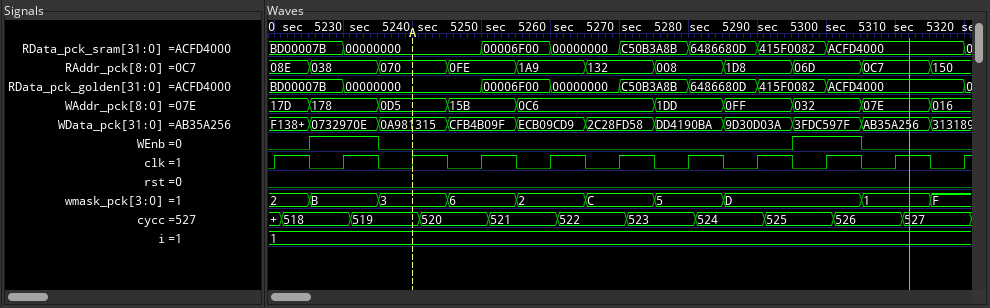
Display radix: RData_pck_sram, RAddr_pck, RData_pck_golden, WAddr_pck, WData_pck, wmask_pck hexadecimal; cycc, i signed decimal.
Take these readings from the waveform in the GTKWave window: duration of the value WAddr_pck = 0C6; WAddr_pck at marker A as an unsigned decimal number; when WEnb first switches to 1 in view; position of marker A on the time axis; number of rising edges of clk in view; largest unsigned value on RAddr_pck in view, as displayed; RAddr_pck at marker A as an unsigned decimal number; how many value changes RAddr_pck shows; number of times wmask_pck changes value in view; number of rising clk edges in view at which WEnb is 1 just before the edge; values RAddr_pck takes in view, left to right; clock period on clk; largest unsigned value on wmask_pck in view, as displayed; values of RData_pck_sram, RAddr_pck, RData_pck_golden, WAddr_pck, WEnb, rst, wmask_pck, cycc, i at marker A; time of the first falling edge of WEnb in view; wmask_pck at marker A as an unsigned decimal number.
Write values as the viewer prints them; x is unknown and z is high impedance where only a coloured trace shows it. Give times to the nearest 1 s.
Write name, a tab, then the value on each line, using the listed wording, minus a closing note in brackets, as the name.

duration of the value WAddr_pck = 0C6	20 s
WAddr_pck at marker A as an unsigned decimal number	213
when WEnb first switches to 1 in view	5225 s
position of marker A on the time axis	5240 s
number of rising edges of clk in view	11
largest unsigned value on RAddr_pck in view, as displayed	1D8
RAddr_pck at marker A as an unsigned decimal number	112
how many value changes RAddr_pck shows	10
number of times wmask_pck changes value in view	9
number of rising clk edges in view at which WEnb is 1 just before the edge	2
values RAddr_pck takes in view, left to right	08E, 038, 070, 0FE, 1A9, 132, 008, 1D8, 06D, 0C7, 150
clock period on clk	10 s
largest unsigned value on wmask_pck in view, as displayed	F
values of RData_pck_sram, RAddr_pck, RData_pck_golden, WAddr_pck, WEnb, rst, wmask_pck, cycc, i at marker A	RData_pck_sram=00000000, RAddr_pck=070, RData_pck_golden=00000000, WAddr_pck=0D5, WEnb=0, rst=0, wmask_pck=3, cycc=519, i=1
time of the first falling edge of WEnb in view	5235 s
wmask_pck at marker A as an unsigned decimal number	3
